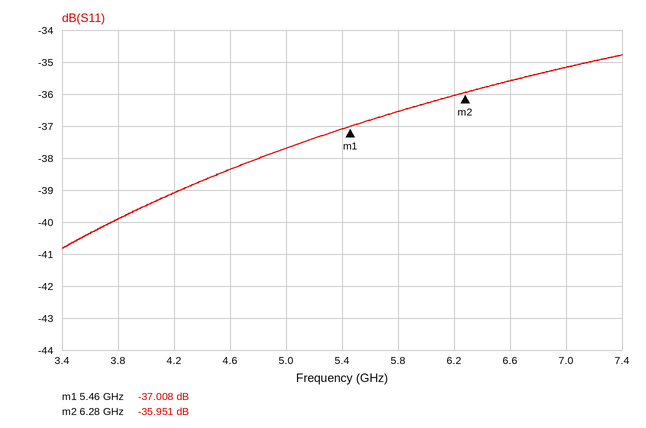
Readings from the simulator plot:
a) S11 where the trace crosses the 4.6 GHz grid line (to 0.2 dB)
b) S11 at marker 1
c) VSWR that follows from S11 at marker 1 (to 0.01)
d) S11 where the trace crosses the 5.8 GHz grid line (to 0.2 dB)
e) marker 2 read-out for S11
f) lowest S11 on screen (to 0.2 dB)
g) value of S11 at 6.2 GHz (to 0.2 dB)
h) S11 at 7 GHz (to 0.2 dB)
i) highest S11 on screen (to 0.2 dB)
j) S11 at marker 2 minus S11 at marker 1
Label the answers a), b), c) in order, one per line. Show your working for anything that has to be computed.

a) -38.4 dB
b) -37.008 dB
c) (1 + 0.0141)/(1 − 0.0141) ≈ 1.03
d) -36.6 dB
e) -35.951 dB
f) -40.8 dB
g) -36.0 dB
h) -35.2 dB
i) -34.8 dB
j) -35.951 − (-37.008) = 1.057 dB
